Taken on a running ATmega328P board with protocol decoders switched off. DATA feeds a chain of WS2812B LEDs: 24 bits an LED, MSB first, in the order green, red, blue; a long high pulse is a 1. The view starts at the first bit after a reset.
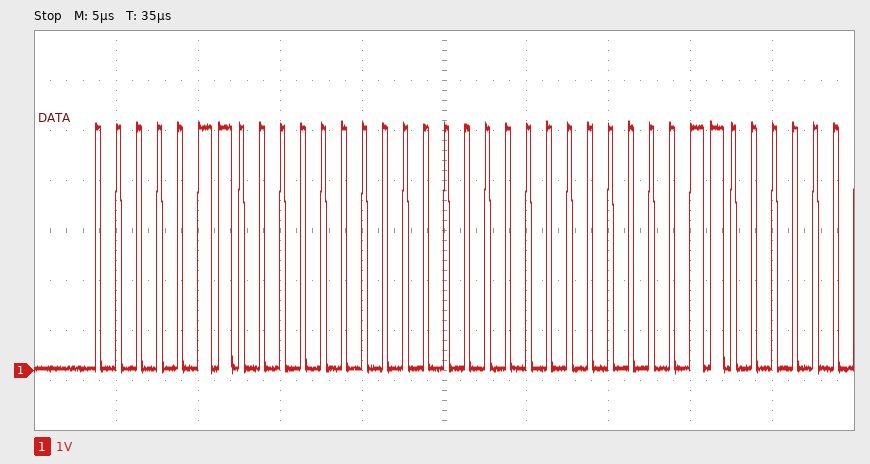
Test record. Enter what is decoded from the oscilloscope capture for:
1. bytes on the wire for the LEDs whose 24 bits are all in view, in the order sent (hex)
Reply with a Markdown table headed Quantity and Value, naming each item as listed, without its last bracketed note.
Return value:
| Quantity | Value |
|---|---|
| bytes on the wire for the LEDs whose 24 bits are all in view, in the order sent | 06 00 00 |
